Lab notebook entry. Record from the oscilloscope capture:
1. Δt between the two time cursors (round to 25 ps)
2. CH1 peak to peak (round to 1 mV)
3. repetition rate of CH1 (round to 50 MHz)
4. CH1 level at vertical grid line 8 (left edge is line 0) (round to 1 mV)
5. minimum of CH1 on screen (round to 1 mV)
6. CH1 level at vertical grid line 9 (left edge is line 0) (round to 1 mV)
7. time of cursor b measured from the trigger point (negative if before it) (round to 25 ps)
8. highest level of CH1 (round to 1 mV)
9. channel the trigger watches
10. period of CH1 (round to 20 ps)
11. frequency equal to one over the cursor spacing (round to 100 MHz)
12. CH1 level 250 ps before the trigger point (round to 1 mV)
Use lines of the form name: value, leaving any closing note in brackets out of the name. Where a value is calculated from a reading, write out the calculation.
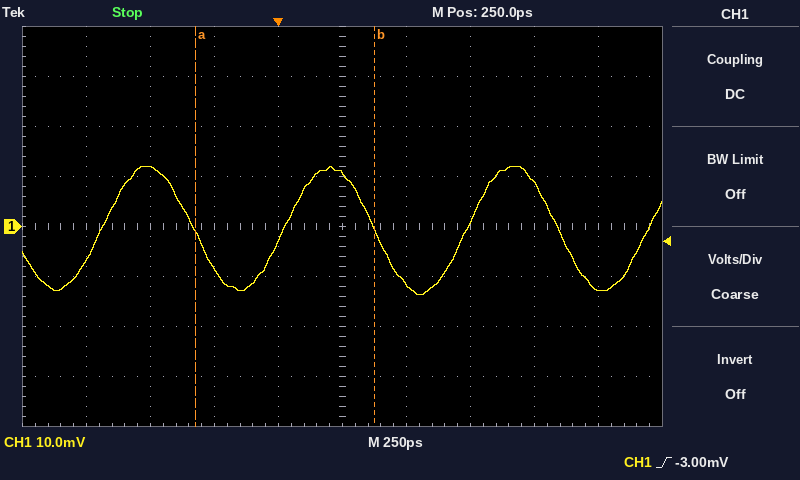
Δt between the two time cursors: 700 ps
CH1 peak to peak: 12 mV − (-14 mV) = 26 mV
repetition rate of CH1: 1 / 720 ps ≈ 1.39 GHz, so 1.40 GHz to the nearest 50 MHz
CH1 level at vertical grid line 8 (left edge is line 0): 9 mV
minimum of CH1 on screen: -14 mV
CH1 level at vertical grid line 9 (left edge is line 0): -13 mV
time of cursor b measured from the trigger point (negative if before it): +375 ps
highest level of CH1: 12 mV
channel the trigger watches: CH1
period of CH1: 720 ps
frequency equal to one over the cursor spacing: 1 / 700 ps ≈ 1.4 GHz
CH1 level 250 ps before the trigger point: -8 mV
